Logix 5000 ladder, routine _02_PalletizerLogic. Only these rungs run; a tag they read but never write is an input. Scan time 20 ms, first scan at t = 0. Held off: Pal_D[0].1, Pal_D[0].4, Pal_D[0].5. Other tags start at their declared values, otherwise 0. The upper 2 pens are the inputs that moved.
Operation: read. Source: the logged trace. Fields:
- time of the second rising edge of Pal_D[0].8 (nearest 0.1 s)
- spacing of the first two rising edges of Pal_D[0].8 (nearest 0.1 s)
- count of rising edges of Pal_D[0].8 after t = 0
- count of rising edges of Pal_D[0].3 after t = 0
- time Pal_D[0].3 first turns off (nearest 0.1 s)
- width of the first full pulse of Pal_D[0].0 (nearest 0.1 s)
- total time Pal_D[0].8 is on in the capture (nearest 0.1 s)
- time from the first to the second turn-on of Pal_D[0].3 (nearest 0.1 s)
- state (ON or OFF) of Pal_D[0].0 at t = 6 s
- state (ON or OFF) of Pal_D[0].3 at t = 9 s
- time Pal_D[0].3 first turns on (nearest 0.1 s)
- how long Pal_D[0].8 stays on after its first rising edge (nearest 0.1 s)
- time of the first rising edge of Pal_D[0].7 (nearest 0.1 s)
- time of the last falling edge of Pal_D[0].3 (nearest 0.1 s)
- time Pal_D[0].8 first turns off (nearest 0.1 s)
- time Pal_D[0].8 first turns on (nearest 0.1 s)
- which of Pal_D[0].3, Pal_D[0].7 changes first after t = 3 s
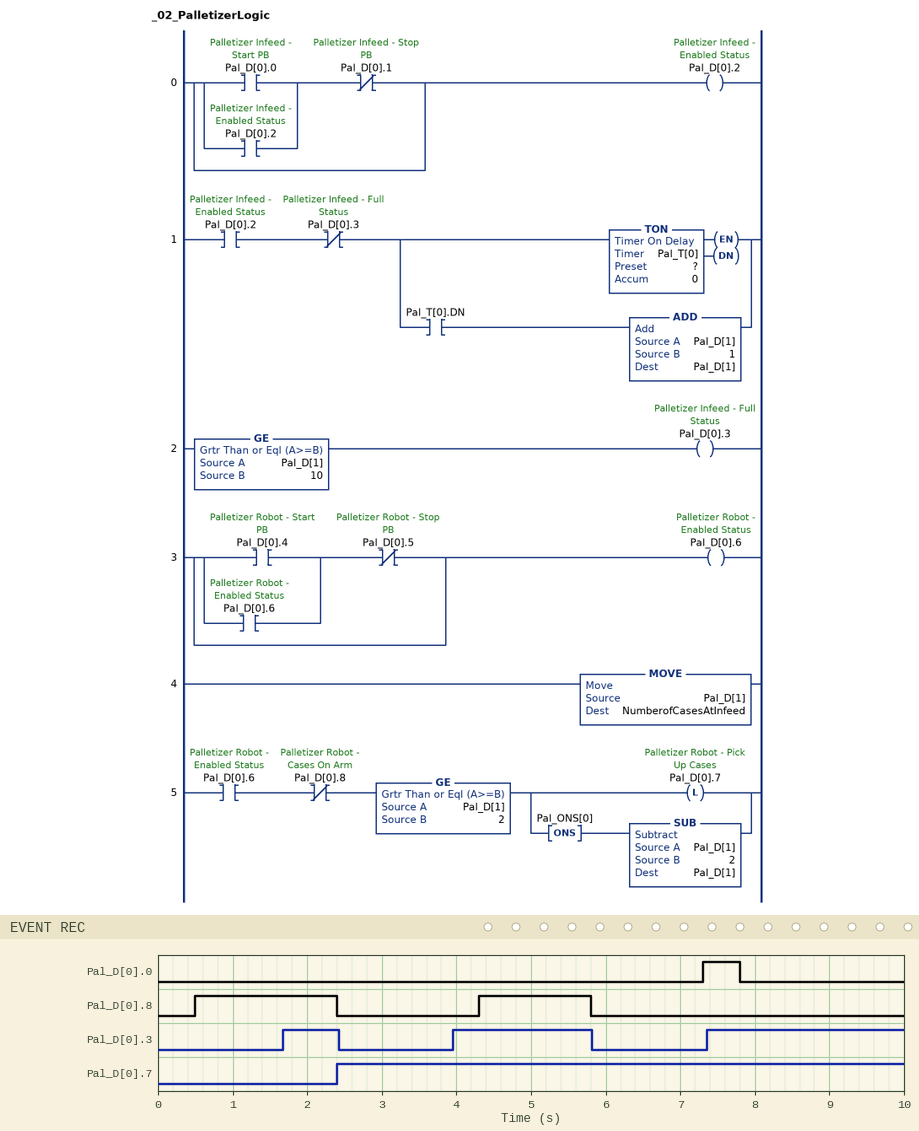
4.3 s
3.8 s
2
3
2.4 s
0.5 s
3.4 s
2.3 s
OFF
ON
1.7 s
1.9 s
2.4 s
5.8 s
2.4 s
0.5 s
Pal_D[0].3
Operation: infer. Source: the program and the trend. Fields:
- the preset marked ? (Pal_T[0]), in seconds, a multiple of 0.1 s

1.5 s
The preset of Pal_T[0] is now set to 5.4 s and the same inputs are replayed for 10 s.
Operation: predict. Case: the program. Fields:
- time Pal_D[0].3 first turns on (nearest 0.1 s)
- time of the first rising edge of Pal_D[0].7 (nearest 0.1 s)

5.6 s
5.8 s
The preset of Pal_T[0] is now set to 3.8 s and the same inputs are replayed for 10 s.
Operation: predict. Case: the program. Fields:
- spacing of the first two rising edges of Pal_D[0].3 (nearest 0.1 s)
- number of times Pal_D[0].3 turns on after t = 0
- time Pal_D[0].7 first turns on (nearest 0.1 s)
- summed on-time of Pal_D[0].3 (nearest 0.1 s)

5.2 s
2
3.8 s
1.7 s
